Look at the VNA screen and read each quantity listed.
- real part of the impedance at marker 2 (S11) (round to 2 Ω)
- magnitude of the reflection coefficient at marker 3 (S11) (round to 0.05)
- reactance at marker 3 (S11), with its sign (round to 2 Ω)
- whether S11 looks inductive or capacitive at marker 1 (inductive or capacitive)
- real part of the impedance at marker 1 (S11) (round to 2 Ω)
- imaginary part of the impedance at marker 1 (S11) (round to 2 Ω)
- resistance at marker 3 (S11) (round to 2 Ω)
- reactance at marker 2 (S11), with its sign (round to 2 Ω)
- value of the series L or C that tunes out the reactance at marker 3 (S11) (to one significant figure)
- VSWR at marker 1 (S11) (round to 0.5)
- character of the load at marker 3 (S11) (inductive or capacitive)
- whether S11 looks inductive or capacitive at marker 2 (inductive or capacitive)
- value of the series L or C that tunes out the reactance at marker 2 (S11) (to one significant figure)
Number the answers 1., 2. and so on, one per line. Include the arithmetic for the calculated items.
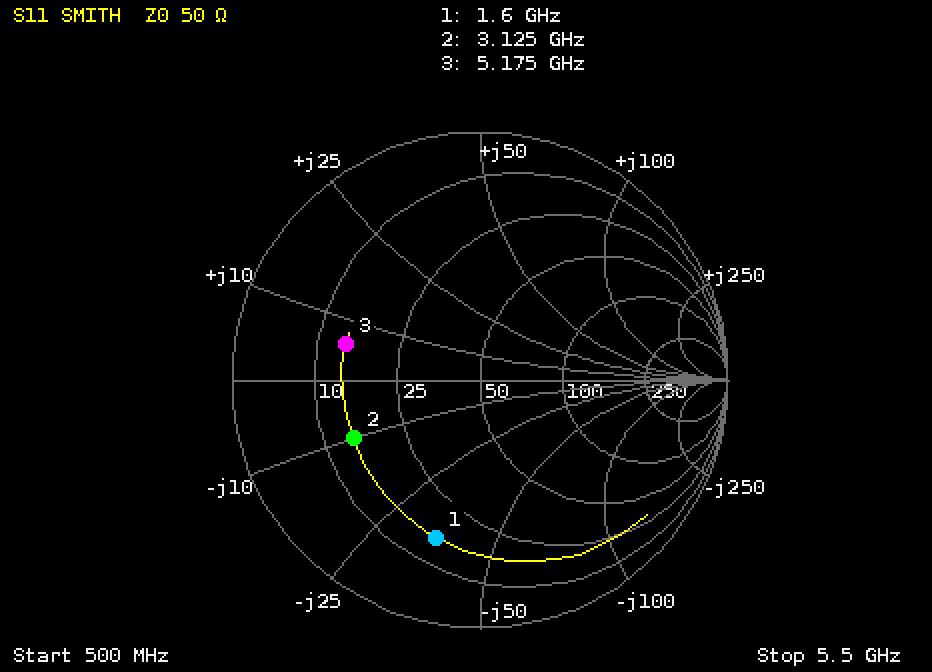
1. 14 Ω
2. 0.55
3. +6 Ω
4. capacitive
5. 16 Ω
6. -36 Ω
7. 14 Ω
8. -10 Ω
9. C = 1/(2π × 5.175 GHz × 6 Ω) ≈ 5 pF
10. 5.0
11. inductive
12. capacitive
13. L = 10 Ω/(2π × 3.125 GHz) ≈ 509 pH, so 500 pH to one significant figure
